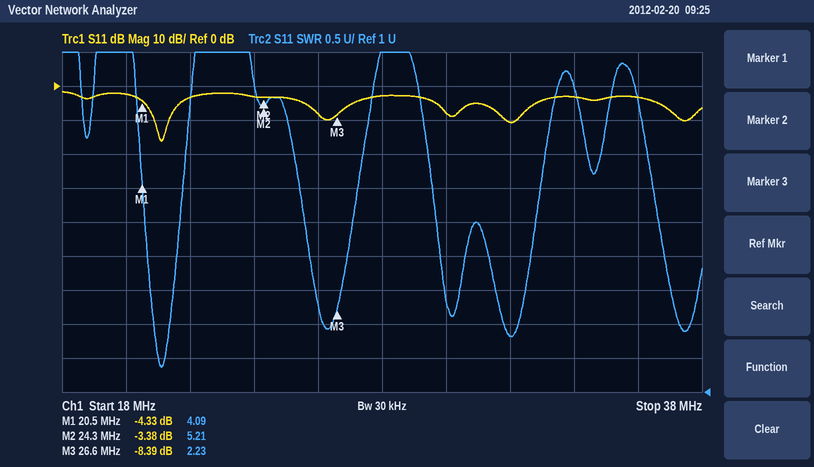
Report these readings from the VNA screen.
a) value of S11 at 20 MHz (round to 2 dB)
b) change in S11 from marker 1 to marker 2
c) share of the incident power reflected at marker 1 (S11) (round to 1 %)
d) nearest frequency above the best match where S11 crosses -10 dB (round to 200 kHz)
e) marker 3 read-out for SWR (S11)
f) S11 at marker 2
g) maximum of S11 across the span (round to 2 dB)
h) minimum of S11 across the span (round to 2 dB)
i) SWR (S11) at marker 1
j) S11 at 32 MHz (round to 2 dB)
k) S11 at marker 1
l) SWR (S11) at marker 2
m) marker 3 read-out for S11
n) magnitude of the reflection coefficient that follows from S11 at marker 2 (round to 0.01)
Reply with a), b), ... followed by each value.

a) -2 dB
b) 0.95 dB
c) 37 %
d) 21.4 MHz
e) 2.23
f) -3.38 dB
g) -2 dB
h) -16 dB
i) 4.09
j) -10 dB
k) -4.33 dB
l) 5.21
m) -8.39 dB
n) 0.68
